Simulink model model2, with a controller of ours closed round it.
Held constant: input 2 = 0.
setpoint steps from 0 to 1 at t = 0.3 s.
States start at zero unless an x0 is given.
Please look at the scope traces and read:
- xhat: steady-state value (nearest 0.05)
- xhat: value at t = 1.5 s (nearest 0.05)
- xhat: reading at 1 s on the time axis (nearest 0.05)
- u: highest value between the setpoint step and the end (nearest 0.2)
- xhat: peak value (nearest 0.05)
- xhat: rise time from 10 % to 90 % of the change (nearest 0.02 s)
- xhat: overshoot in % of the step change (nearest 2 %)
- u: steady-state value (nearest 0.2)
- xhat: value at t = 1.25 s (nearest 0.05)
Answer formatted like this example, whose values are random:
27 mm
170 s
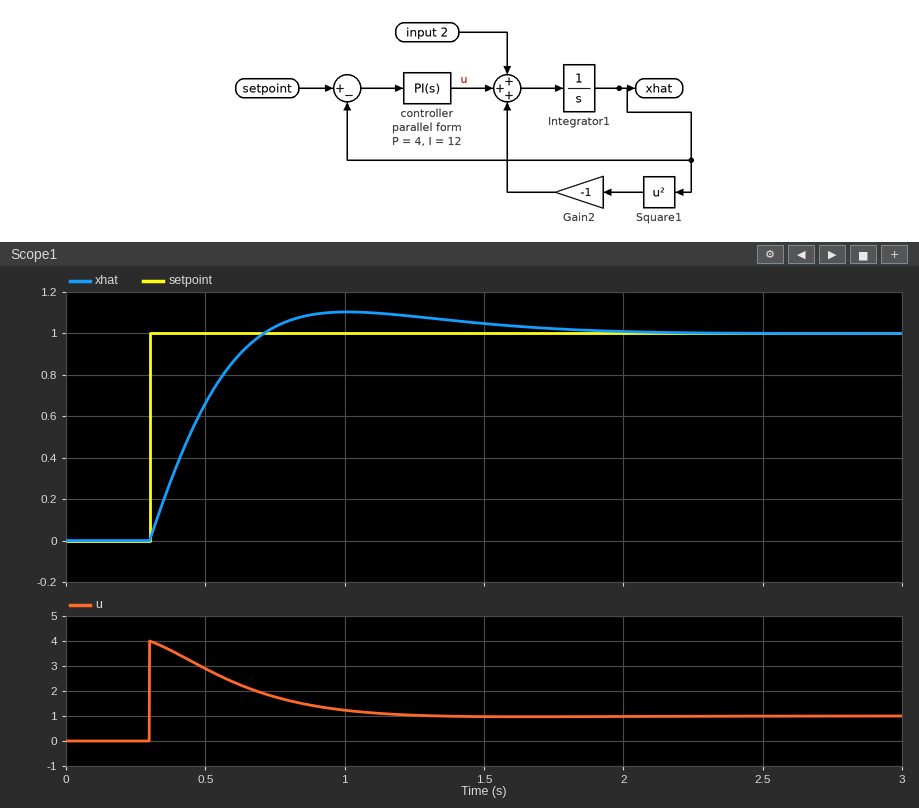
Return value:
1.00
1.05
1.10
4.0
1.10
0.30 s
10 %
1.0
1.10
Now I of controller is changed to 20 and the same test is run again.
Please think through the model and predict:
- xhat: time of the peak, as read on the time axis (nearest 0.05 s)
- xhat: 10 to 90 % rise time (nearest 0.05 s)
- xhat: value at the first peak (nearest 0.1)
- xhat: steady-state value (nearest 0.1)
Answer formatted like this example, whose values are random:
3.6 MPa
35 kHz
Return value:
0.85 s
0.25 s
1.2
1.0
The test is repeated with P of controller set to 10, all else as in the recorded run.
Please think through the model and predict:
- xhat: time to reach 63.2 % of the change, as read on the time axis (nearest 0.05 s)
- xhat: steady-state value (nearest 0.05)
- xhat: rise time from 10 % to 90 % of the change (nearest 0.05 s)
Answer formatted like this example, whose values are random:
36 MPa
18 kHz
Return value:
0.40 s
1.00
0.20 s
